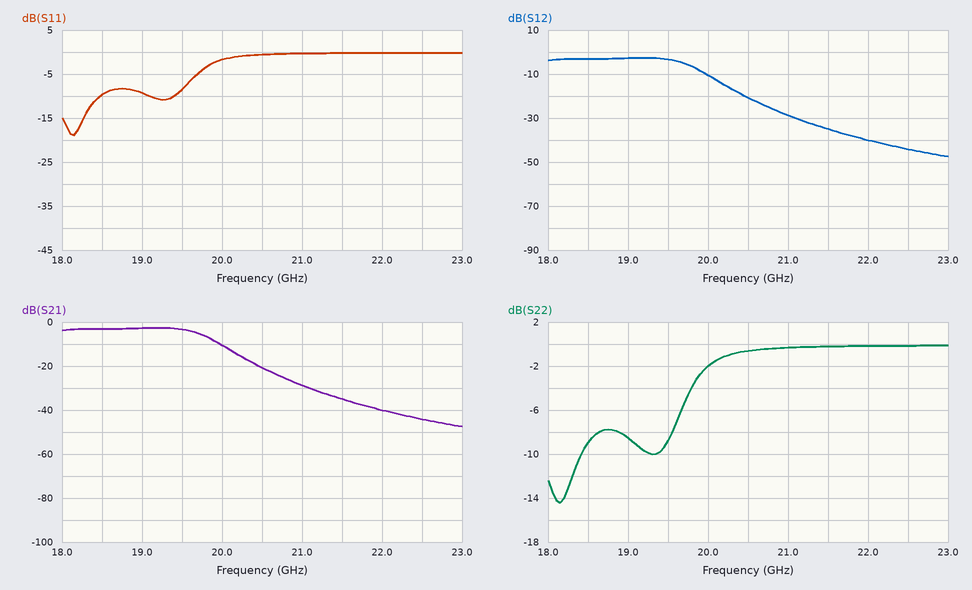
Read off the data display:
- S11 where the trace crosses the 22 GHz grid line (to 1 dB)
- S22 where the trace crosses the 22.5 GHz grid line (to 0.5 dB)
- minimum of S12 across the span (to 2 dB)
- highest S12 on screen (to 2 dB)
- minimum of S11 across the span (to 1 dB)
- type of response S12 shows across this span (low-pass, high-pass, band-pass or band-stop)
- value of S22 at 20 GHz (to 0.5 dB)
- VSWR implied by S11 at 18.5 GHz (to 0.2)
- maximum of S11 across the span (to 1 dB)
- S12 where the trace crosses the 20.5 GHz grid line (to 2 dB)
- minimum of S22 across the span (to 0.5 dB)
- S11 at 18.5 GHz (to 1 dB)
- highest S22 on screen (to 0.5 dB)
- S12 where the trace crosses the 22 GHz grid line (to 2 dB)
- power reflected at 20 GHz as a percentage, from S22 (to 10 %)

0 dB
0.0 dB
-48 dB
-2 dB
-19 dB
low-pass
-2.0 dB
2.0
0 dB
-20 dB
-14.5 dB
-10 dB
0.0 dB
-40 dB
60 %
